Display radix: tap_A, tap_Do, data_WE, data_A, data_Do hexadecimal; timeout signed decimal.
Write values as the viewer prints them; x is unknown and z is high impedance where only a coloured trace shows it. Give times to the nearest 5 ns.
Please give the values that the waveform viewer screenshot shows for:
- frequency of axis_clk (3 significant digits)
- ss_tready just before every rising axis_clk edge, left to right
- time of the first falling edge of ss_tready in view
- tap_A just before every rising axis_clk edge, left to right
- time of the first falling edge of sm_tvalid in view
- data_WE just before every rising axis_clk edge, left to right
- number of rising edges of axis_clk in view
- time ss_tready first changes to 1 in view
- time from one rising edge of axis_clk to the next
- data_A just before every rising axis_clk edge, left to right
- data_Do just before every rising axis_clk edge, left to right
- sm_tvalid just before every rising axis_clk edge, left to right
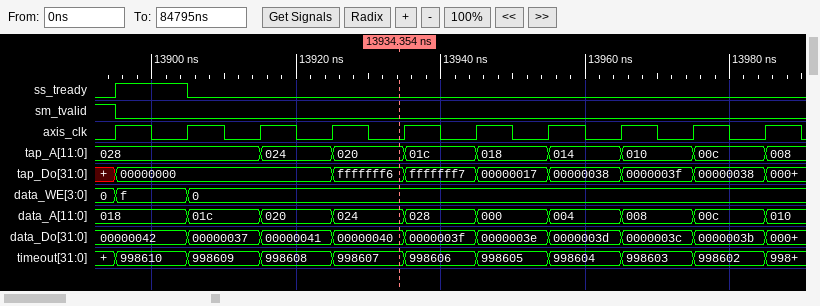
100 MHz
0 1 0 0 0 0 0 0 0 0
13905 ns
028, 028, 028, 024, 020, 01c, 018, 014, 010, 00c
13895 ns
0, f, 0, 0, 0, 0, 0, 0, 0, 0
10
13895 ns
10 ns
018, 018, 01c, 020, 024, 028, 000, 004, 008, 00c
00000042, 00000042, 00000037, 00000041, 00000040, 0000003f, 0000003e, 0000003d, 0000003c, 0000003b
1 0 0 0 0 0 0 0 0 0
